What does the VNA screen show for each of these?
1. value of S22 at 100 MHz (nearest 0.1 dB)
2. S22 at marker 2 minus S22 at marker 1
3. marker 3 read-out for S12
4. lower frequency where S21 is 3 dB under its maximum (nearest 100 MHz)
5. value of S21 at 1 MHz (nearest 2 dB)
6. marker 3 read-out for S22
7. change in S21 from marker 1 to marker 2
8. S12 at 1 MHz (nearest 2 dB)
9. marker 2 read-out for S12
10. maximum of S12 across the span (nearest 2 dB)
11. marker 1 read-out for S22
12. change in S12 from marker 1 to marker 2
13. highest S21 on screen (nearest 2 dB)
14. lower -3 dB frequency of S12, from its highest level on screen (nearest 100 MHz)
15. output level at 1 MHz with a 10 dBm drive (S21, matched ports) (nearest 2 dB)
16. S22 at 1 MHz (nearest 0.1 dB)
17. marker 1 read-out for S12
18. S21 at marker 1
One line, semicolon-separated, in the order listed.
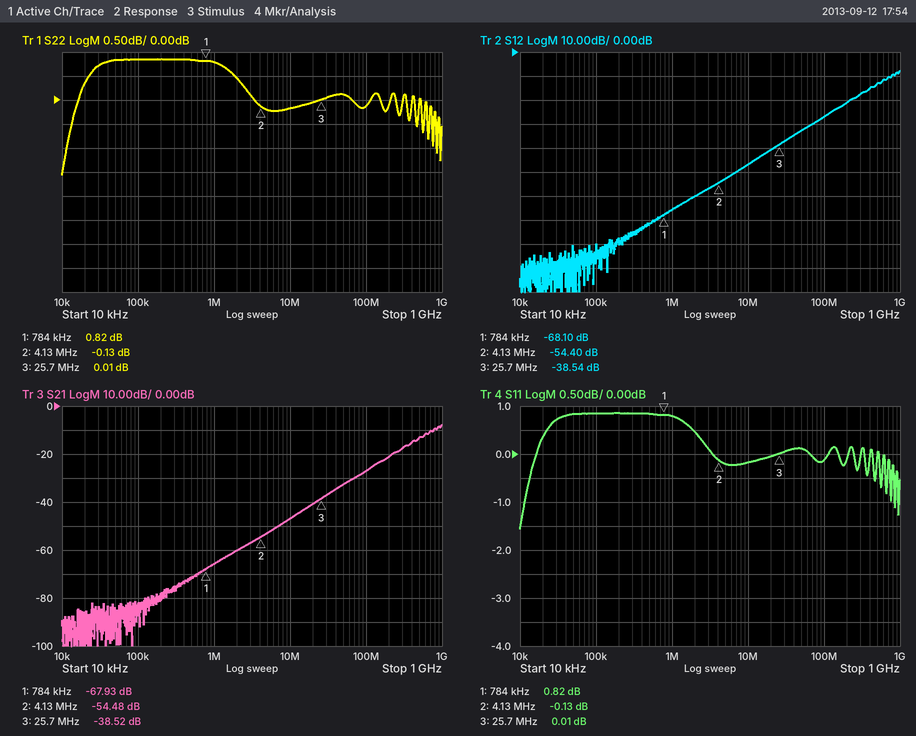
-0.1 dB; -0.95 dB; -38.54 dB; 700 MHz; -66 dB; 0.01 dB; 13.45 dB; -66 dB; -54.40 dB; -8 dB; 0.82 dB; 13.70 dB; -8 dB; 700 MHz; -56 dBm; 0.8 dB; -68.10 dB; -67.93 dB
